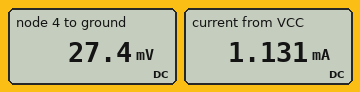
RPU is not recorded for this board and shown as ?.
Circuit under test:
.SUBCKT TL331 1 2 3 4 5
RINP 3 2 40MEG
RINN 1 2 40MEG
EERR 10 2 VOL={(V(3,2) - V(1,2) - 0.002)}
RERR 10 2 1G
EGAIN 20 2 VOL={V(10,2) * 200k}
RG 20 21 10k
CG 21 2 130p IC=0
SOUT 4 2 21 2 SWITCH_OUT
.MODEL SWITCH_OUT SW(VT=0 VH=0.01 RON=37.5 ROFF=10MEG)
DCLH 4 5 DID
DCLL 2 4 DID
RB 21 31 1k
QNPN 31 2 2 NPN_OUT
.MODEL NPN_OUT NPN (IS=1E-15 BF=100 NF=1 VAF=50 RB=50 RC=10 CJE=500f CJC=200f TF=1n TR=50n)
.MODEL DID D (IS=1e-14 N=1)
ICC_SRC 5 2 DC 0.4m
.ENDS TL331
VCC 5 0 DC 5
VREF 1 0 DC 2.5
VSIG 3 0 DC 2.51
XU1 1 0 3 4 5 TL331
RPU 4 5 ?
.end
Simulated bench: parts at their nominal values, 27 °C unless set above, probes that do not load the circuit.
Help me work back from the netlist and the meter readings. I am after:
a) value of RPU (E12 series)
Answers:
6.8 kΩ
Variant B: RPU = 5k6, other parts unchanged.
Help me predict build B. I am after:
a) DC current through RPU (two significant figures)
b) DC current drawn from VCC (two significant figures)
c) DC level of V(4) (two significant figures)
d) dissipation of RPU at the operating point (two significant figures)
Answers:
890 µA
1.3 mA
33 mV
4.4 mW
